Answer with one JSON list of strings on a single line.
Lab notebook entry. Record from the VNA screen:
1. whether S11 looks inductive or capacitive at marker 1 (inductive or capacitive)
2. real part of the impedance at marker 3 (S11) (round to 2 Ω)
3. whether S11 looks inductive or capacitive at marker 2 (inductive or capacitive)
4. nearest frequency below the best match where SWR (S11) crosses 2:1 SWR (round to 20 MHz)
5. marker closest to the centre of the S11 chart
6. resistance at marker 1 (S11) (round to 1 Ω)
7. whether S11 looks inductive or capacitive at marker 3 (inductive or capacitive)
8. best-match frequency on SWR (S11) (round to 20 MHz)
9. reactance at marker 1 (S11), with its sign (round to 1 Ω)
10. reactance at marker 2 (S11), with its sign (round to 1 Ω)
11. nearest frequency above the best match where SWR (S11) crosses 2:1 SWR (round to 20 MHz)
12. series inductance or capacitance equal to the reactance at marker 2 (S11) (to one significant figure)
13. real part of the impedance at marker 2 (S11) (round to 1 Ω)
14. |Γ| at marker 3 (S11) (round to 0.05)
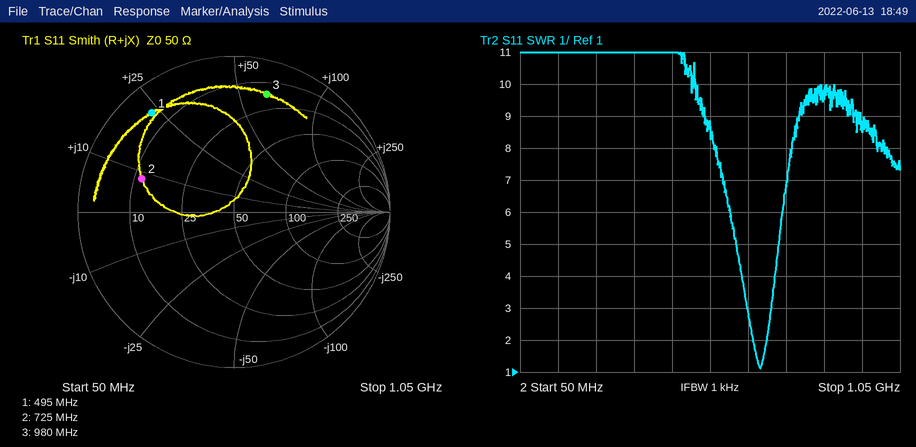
["inductive", "16 Ω", "inductive", "660 MHz", "marker 2", "6 Ω", "inductive", "680 MHz", "+23 Ω", "+8 Ω", "700 MHz", "2 nH", "12 Ω", "0.80"]
